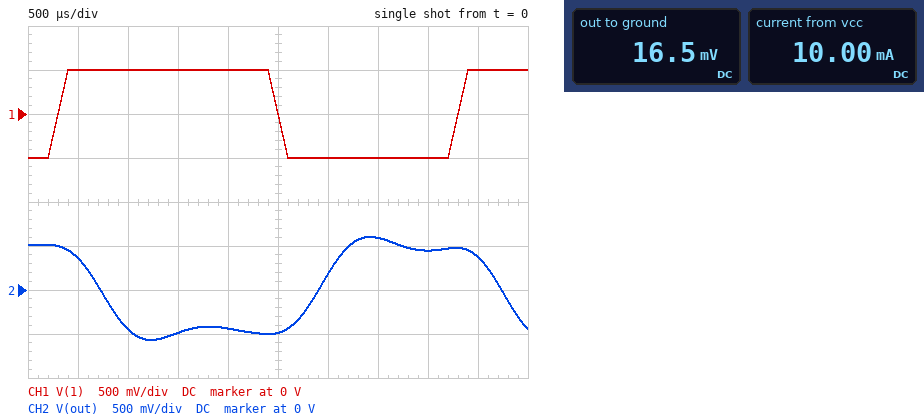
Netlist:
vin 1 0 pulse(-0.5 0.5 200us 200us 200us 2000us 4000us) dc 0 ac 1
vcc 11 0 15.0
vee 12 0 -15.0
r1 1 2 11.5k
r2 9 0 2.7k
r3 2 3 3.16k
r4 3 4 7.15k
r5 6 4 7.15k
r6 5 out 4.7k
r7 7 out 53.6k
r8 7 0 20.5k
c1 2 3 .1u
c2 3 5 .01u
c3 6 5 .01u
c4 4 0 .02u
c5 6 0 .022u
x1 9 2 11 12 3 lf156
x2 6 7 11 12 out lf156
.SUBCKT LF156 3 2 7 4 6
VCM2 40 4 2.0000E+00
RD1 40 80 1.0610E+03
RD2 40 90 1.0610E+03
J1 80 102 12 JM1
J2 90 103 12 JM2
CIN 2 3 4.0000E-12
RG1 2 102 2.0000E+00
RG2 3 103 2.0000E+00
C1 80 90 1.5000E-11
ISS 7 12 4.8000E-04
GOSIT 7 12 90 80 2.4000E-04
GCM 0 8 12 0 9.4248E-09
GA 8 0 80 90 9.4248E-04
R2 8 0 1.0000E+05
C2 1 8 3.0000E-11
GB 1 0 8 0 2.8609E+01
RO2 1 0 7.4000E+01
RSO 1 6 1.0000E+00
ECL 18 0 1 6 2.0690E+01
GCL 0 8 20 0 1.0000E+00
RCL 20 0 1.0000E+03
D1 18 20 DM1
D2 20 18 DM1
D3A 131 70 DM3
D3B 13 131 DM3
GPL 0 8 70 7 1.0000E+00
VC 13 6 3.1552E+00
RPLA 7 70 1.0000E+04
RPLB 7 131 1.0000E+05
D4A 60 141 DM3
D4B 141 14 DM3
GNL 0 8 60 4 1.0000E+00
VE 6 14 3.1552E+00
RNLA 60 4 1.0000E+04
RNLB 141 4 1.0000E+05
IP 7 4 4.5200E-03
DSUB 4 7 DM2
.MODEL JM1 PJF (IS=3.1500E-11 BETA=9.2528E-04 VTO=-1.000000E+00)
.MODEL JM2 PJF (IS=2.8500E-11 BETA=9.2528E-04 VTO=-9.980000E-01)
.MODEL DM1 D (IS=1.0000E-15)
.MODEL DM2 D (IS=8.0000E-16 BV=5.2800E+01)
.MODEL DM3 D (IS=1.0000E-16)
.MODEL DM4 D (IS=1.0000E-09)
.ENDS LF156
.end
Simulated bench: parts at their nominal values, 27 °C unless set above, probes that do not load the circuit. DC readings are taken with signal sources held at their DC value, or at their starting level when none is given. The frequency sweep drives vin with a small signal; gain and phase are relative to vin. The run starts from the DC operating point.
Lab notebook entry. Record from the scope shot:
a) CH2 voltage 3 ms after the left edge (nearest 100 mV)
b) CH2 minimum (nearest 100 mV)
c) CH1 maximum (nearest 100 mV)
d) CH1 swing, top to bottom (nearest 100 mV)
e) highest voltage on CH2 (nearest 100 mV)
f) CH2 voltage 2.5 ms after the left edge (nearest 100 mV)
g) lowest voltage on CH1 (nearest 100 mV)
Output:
200 mV
-600 mV
500 mV
1.0 V
600 mV
-500 mV
-500 mV
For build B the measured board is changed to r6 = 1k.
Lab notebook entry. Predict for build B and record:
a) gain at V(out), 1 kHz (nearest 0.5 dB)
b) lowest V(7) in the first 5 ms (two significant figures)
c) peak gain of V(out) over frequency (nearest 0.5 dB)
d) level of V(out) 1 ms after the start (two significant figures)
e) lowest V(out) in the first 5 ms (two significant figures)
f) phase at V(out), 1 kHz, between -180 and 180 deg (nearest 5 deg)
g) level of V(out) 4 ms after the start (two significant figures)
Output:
-6.5 dB
-140 mV
1.5 dB
-290 mV
-500 mV
90 deg
490 mV
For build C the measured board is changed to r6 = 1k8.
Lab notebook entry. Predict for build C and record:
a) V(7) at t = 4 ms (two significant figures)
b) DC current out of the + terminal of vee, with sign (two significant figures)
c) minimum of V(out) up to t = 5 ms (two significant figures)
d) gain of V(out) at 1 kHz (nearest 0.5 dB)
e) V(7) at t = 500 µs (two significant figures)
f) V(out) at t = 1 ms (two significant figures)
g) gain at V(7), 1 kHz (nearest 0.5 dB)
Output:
140 mV
-10 mA
-490 mV
-4.0 dB
87 mV
-380 mV
-15.0 dB
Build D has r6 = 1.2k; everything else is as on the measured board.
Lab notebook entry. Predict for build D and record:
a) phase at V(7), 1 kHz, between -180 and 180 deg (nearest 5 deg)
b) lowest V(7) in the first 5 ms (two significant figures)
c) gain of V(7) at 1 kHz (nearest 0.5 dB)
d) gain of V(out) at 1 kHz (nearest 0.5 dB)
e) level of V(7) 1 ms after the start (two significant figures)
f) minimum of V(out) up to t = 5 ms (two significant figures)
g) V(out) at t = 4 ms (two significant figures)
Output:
85 deg
-140 mV
-17.0 dB
-6.0 dB
-79 mV
-490 mV
520 mV
